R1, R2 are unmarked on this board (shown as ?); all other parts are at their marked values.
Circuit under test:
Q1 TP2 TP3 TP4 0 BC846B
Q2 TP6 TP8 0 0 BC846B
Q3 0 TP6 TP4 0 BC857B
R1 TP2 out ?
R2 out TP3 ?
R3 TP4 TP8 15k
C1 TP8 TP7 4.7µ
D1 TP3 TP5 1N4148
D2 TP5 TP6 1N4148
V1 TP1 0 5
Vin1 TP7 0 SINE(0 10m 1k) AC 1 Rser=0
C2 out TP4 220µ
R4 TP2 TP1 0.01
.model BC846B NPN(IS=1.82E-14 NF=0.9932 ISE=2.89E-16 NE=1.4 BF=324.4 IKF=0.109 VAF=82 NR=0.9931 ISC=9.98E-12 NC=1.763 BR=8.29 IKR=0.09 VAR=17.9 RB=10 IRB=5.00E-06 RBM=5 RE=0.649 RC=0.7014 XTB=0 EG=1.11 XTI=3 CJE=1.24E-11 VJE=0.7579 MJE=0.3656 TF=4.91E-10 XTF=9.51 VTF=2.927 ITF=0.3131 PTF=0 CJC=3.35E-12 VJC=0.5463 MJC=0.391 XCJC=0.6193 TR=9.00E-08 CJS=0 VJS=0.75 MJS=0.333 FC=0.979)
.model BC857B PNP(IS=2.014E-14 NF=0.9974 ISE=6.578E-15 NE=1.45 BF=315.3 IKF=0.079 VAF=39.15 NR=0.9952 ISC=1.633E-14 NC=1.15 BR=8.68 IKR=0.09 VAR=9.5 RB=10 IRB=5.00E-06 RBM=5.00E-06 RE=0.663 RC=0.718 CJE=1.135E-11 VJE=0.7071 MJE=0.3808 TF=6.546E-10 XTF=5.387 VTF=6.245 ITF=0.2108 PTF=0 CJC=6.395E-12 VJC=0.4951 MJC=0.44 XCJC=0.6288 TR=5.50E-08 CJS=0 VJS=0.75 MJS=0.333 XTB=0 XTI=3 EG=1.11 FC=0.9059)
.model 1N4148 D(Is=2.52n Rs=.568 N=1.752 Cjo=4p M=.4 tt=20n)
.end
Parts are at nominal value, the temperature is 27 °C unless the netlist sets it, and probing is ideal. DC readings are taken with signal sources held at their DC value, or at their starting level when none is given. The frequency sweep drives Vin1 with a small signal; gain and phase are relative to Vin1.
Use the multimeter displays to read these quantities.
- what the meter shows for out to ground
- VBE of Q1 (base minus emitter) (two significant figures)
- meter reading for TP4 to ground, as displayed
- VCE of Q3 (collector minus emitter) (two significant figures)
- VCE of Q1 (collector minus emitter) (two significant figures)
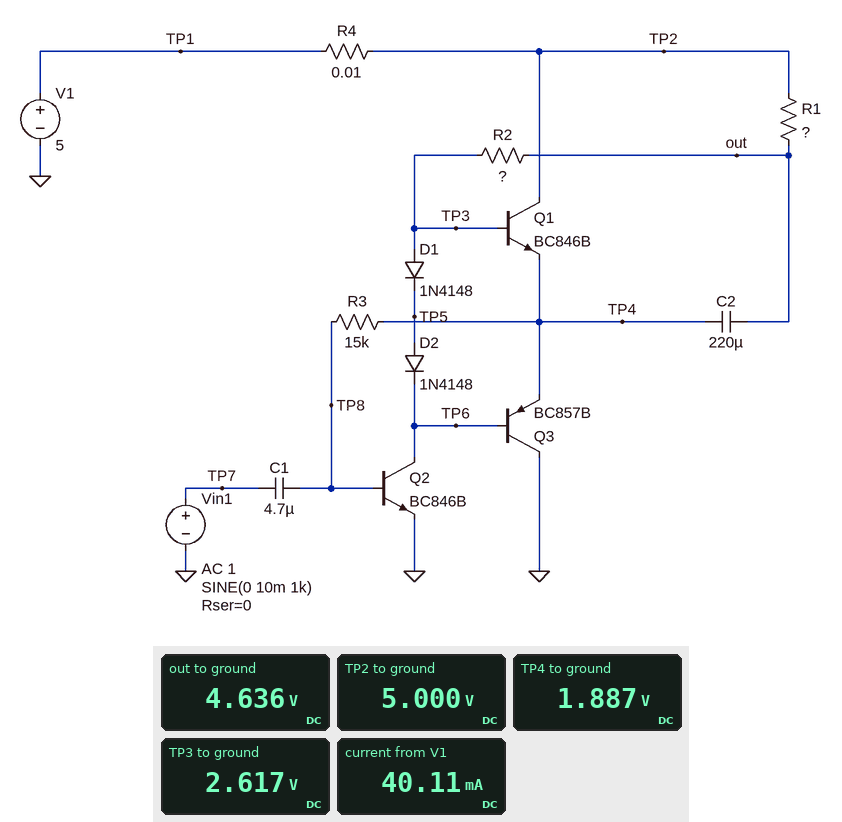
4.636 V
730 mV
1.887 V
-1.9 V
3.1 V
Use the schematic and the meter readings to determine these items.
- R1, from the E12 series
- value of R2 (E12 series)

18 Ω
100 Ω
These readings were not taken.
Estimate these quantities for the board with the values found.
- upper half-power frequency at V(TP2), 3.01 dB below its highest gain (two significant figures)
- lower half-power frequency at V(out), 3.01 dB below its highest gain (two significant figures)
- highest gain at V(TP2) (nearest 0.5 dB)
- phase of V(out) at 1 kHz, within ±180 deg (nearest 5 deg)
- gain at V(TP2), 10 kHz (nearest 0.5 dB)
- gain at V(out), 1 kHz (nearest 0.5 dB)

3.1 MHz
1.4 kHz
-18.0 dB
-125 deg
-18.0 dB
48.0 dB
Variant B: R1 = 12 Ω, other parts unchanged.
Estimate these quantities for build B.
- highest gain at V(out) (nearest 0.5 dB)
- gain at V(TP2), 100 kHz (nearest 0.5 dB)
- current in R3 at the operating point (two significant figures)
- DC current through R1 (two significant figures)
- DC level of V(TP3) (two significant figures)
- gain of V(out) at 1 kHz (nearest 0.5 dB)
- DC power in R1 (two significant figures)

50.0 dB
-17.0 dB
80 µA
21 mA
2.7 V
46.5 dB
5.2 mW
